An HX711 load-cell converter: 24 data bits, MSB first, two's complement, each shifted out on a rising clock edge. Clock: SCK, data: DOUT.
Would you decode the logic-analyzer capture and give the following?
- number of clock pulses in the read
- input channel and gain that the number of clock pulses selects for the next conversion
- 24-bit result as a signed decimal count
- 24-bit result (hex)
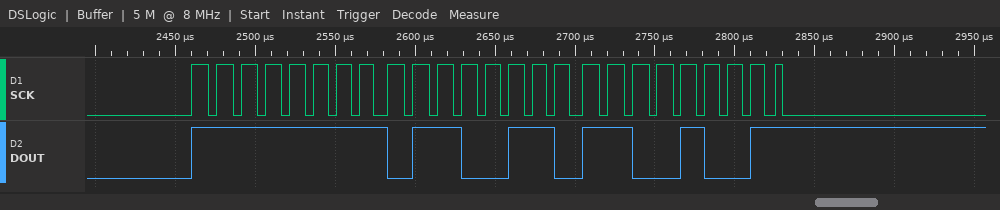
25
channel A, gain 128
-39223
0xFF66C9
